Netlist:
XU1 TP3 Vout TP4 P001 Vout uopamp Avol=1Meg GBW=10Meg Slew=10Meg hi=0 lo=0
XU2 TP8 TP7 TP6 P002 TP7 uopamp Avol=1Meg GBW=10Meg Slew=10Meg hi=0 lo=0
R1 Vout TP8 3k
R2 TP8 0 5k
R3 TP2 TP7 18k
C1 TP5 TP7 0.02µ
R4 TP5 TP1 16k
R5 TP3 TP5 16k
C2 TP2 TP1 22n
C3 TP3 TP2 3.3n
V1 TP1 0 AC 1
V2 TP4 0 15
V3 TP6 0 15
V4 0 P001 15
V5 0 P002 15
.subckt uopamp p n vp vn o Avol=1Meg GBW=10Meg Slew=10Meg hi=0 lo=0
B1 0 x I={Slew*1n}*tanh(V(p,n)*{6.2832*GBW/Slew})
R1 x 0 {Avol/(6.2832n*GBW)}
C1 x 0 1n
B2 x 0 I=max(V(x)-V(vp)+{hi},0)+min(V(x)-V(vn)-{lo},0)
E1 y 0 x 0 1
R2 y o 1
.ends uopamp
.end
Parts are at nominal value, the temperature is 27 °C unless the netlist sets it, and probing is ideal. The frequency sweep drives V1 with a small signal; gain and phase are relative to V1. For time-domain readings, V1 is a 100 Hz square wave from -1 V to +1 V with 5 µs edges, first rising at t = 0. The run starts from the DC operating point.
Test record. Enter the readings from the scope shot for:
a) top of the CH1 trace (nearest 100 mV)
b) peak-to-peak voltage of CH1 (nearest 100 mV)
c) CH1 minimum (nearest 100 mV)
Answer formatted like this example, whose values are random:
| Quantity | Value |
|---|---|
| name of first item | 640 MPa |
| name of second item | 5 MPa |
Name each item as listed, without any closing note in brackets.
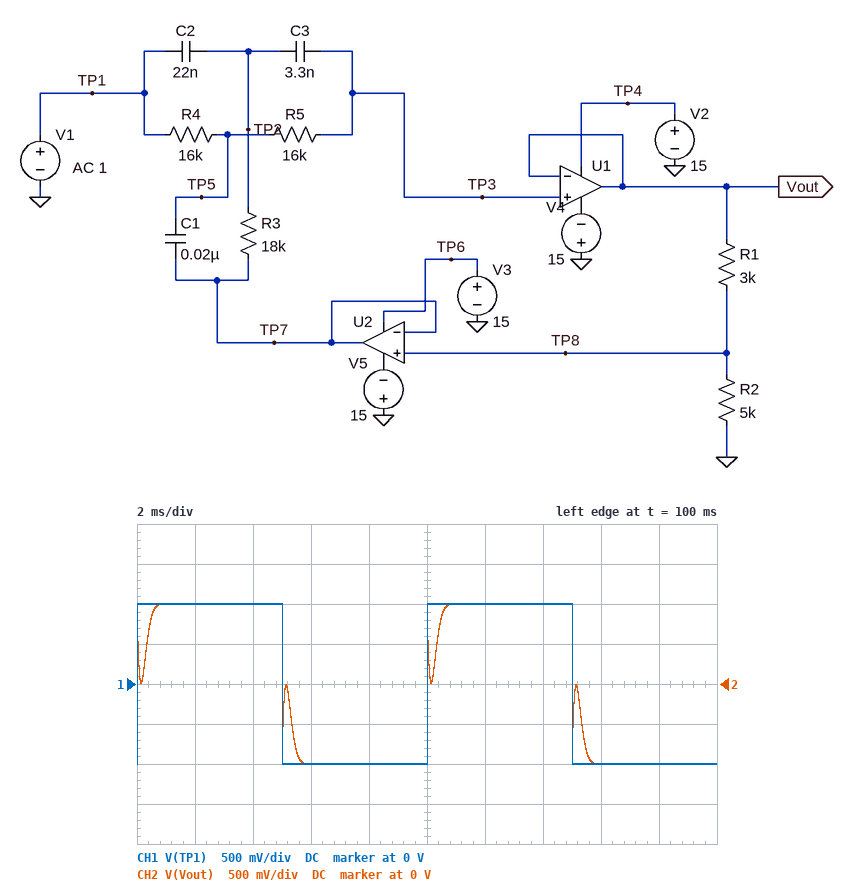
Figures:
| Quantity | Value |
|---|---|
| top of the CH1 trace | 1.0 V |
| peak-to-peak voltage of CH1 | 2.0 V |
| CH1 minimum | -1.0 V |
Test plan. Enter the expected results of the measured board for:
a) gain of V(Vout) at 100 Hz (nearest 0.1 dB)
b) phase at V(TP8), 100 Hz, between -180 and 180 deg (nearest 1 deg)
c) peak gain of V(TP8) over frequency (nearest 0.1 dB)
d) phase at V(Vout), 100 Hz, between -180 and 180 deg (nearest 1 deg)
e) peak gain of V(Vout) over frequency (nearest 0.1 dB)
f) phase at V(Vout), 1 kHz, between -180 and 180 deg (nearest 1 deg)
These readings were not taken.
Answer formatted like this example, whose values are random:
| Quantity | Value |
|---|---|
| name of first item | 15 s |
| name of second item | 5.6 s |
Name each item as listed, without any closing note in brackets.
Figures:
| Quantity | Value |
|---|---|
| gain of V(Vout) at 100 Hz | -0.1 dB |
| phase at V(TP8), 100 Hz, between -180 and 180 deg | -6 deg |
| peak gain of V(TP8) over frequency | -4.1 dB |
| phase at V(Vout), 100 Hz, between -180 and 180 deg | -6 deg |
| peak gain of V(Vout) over frequency | 0 dB |
| phase at V(Vout), 1 kHz, between -180 and 180 deg | -26 deg |
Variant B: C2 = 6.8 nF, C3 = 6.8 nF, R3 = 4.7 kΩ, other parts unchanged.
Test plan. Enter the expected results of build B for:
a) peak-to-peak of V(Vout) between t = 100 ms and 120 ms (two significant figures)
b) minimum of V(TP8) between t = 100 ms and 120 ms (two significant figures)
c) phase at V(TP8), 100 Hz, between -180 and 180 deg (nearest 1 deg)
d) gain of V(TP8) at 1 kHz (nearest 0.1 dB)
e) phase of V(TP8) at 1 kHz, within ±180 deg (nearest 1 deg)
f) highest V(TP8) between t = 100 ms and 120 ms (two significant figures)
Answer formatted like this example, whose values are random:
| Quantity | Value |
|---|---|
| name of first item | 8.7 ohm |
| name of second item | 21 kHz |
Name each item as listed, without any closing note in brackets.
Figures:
| Quantity | Value |
|---|---|
| peak-to-peak of V(Vout) between t = 100 ms and 120 ms | 2.1 V |
| minimum of V(TP8) between t = 100 ms and 120 ms | -650 mV |
| phase at V(TP8), 100 Hz, between -180 and 180 deg | -7 deg |
| gain of V(TP8) at 1 kHz | -9.6 dB |
| phase of V(TP8) at 1 kHz, within ±180 deg | -84 deg |
| highest V(TP8) between t = 100 ms and 120 ms | 650 mV |
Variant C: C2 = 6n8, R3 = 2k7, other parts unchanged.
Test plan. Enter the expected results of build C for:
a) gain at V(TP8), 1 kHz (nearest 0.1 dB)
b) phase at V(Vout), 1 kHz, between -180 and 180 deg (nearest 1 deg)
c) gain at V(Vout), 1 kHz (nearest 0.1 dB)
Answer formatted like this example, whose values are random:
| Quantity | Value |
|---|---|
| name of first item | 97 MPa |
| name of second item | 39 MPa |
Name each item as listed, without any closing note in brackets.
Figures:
| Quantity | Value |
|---|---|
| gain at V(TP8), 1 kHz | -6.5 dB |
| phase at V(Vout), 1 kHz, between -180 and 180 deg | -58 deg |
| gain at V(Vout), 1 kHz | -2.4 dB |
